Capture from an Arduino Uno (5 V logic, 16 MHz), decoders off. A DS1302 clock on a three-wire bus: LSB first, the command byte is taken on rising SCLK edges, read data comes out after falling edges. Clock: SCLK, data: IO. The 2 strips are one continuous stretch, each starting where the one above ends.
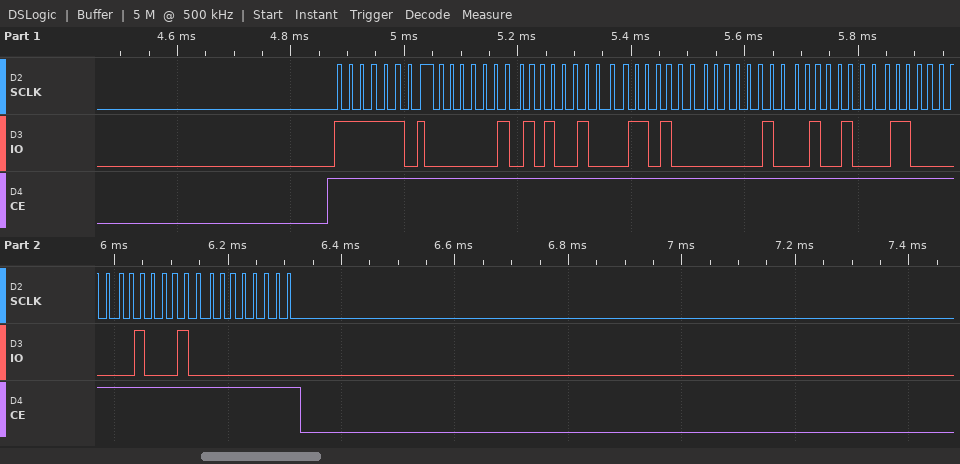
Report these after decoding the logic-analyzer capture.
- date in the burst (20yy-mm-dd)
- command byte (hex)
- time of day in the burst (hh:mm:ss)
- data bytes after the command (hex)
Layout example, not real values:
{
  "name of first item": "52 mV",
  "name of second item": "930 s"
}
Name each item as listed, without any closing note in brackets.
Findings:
{
  "date in the burst": "2022-12-20",
  "command byte": "0xBF",
  "time of day in the burst": "16:25:40",
  "data bytes after the command": "40 25 16 20 12 03 22 00"
}
